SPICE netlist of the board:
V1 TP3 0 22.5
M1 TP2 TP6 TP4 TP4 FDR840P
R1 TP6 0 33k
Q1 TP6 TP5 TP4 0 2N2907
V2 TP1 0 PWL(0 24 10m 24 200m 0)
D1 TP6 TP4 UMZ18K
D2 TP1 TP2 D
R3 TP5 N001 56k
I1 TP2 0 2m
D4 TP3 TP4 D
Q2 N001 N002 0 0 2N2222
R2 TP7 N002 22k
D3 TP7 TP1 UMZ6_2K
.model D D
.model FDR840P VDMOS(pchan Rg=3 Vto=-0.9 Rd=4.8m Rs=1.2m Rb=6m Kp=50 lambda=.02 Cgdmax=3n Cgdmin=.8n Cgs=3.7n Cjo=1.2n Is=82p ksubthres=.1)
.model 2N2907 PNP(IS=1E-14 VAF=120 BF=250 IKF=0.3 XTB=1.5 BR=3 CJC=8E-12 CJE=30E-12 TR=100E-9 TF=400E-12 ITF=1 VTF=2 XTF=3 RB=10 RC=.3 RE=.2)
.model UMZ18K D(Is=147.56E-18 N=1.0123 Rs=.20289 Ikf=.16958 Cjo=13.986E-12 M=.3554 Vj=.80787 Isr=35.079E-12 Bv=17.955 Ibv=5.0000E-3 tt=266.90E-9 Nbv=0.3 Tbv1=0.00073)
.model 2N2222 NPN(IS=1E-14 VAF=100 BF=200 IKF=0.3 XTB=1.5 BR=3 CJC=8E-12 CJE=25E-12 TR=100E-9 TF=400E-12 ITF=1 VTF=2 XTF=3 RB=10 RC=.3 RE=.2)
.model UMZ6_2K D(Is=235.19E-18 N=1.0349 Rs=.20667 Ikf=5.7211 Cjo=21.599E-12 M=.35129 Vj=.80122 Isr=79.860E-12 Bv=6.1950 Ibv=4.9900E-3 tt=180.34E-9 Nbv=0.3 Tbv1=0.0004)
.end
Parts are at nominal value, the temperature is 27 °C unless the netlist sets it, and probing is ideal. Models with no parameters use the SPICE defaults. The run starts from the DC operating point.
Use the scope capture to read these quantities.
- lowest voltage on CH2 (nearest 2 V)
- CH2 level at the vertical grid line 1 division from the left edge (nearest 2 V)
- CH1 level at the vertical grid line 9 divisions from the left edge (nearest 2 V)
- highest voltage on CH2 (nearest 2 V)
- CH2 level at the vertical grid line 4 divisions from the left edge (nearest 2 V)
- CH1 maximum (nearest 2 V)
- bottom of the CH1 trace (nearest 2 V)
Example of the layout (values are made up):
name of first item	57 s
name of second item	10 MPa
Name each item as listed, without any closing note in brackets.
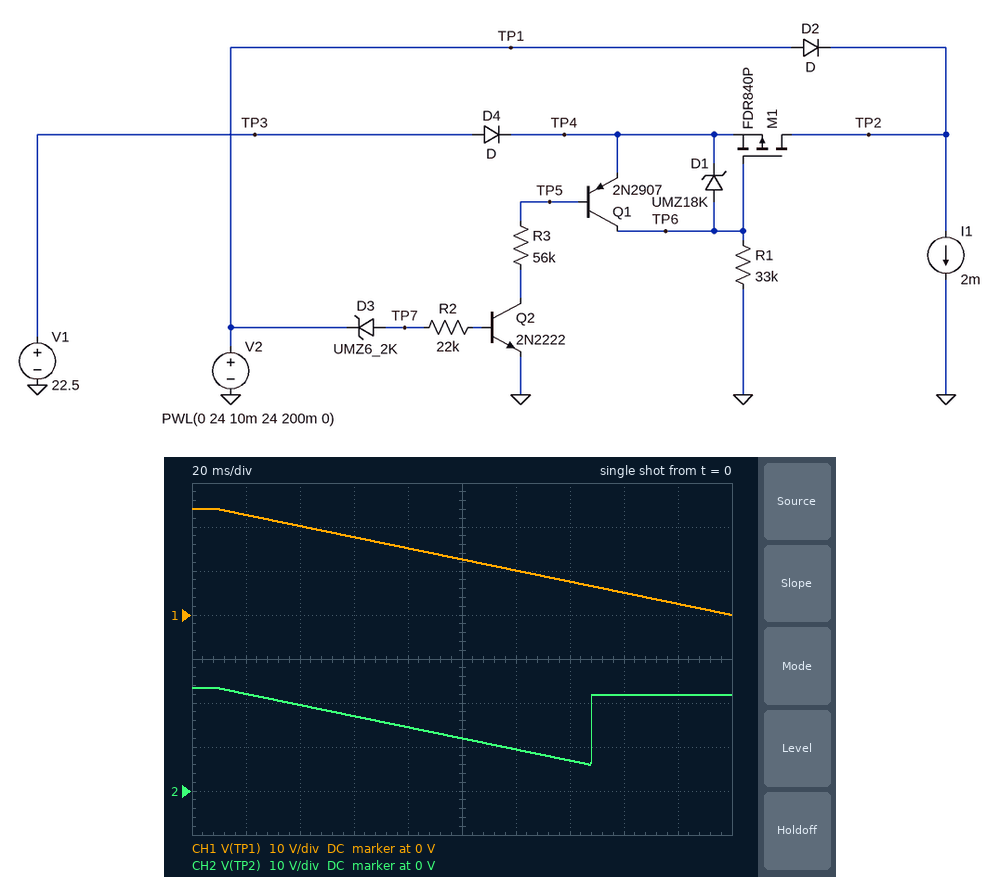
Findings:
lowest voltage on CH2	6 V
CH2 level at the vertical grid line 1 division from the left edge	22 V
CH1 level at the vertical grid line 9 divisions from the left edge	2 V
highest voltage on CH2	24 V
CH2 level at the vertical grid line 4 divisions from the left edge	14 V
CH1 maximum	24 V
bottom of the CH1 trace	0 V
